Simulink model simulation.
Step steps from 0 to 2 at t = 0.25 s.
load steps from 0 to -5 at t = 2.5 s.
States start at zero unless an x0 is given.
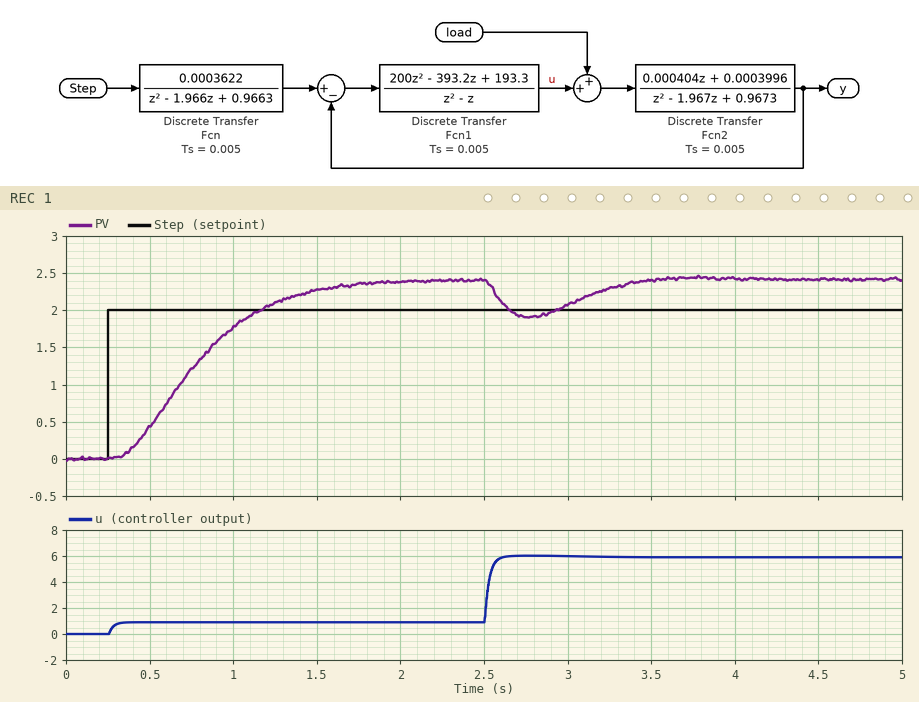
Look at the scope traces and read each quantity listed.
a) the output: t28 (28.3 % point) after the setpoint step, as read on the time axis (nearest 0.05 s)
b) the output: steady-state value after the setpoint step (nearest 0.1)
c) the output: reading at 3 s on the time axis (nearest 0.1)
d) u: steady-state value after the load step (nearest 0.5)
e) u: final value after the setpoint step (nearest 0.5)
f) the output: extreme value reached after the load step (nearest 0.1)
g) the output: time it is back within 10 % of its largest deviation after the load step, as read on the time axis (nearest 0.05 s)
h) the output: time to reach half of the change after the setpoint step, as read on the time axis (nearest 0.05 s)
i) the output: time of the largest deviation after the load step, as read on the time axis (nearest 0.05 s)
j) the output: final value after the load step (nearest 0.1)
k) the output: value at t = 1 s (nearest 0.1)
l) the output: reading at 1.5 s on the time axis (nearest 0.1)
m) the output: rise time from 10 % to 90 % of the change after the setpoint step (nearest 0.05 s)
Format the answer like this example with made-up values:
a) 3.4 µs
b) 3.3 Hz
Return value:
a) 0.60 s
b) 2.4
c) 2.1
d) 6.0
e) 1.0
f) 1.9
g) 3.40 s
h) 0.75 s
i) 2.75 s
j) 2.4
k) 1.8
l) 2.3
m) 0.90 s
